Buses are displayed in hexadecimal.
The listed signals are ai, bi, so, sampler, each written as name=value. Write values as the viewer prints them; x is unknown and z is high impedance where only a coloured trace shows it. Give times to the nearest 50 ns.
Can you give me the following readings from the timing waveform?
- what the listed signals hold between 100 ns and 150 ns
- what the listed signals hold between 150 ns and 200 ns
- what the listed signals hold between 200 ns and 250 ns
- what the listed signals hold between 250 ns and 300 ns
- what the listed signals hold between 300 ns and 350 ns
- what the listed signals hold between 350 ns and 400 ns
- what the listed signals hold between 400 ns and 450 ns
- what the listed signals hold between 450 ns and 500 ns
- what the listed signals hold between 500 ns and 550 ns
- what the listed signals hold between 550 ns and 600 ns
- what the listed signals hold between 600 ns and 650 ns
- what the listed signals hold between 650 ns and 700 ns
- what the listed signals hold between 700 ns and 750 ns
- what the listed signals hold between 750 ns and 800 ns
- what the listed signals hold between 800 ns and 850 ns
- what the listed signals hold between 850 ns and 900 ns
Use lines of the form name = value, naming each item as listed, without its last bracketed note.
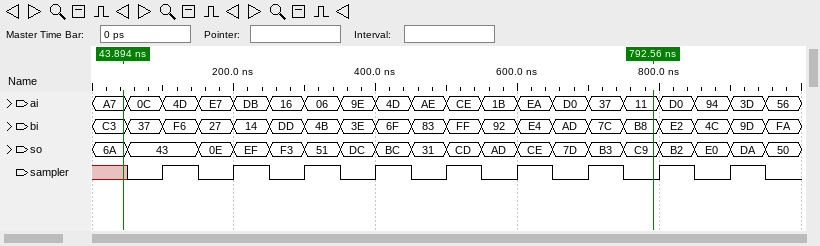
what the listed signals hold between 100 ns and 150 ns = ai=4D, bi=F6, so=43, sampler=1
what the listed signals hold between 150 ns and 200 ns = ai=E7, bi=27, so=0E, sampler=0
what the listed signals hold between 200 ns and 250 ns = ai=DB, bi=14, so=EF, sampler=1
what the listed signals hold between 250 ns and 300 ns = ai=16, bi=DD, so=F3, sampler=0
what the listed signals hold between 300 ns and 350 ns = ai=06, bi=4B, so=51, sampler=1
what the listed signals hold between 350 ns and 400 ns = ai=9E, bi=3E, so=DC, sampler=0
what the listed signals hold between 400 ns and 450 ns = ai=4D, bi=6F, so=BC, sampler=1
what the listed signals hold between 450 ns and 500 ns = ai=AE, bi=83, so=31, sampler=0
what the listed signals hold between 500 ns and 550 ns = ai=CE, bi=FF, so=CD, sampler=1
what the listed signals hold between 550 ns and 600 ns = ai=1B, bi=92, so=AD, sampler=0
what the listed signals hold between 600 ns and 650 ns = ai=EA, bi=E4, so=CE, sampler=1
what the listed signals hold between 650 ns and 700 ns = ai=D0, bi=AD, so=7D, sampler=0
what the listed signals hold between 700 ns and 750 ns = ai=37, bi=7C, so=B3, sampler=1
what the listed signals hold between 750 ns and 800 ns = ai=11, bi=B8, so=C9, sampler=0
what the listed signals hold between 800 ns and 850 ns = ai=D0, bi=E2, so=B2, sampler=1
what the listed signals hold between 850 ns and 900 ns = ai=94, bi=4C, so=E0, sampler=0
